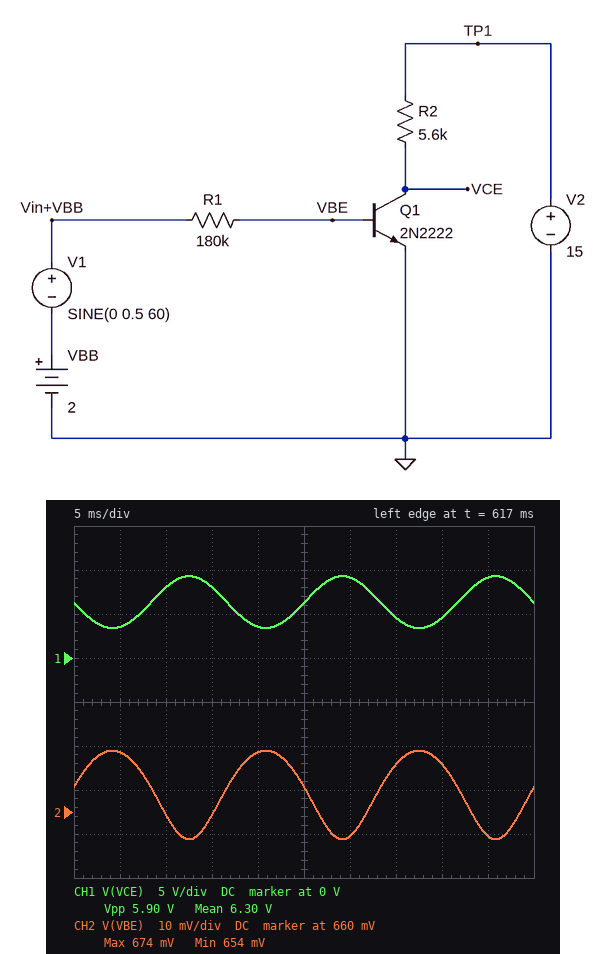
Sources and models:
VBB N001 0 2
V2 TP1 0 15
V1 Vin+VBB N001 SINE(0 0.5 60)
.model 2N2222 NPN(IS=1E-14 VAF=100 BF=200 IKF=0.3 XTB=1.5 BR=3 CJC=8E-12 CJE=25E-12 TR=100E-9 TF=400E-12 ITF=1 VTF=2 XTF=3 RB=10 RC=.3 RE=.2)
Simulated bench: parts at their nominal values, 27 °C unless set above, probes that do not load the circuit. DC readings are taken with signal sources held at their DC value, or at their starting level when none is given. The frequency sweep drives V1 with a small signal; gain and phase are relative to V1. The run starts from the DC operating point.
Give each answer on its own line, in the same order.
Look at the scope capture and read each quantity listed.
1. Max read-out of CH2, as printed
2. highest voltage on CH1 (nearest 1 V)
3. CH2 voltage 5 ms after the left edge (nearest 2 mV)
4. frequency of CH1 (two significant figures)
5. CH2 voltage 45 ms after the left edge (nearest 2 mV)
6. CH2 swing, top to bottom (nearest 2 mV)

674 mV
9 V
674 mV
60 Hz
654 mV
20 mV
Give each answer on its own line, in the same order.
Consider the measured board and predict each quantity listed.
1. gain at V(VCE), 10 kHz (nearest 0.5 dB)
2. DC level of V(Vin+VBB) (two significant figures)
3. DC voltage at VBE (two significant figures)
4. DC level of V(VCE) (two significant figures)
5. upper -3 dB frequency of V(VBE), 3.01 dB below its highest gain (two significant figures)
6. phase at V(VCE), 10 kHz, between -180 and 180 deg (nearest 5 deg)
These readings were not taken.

15.0 dB
2.0 V
670 mV
6.3 V
36 kHz
165 deg
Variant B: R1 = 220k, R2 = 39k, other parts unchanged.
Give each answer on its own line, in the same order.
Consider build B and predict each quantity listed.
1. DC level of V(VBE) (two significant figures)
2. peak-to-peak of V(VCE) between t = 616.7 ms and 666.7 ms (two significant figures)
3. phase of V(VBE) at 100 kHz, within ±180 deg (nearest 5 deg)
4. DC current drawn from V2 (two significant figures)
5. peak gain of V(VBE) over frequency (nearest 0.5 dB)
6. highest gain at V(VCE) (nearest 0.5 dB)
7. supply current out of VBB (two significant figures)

630 mV
29 mV
-10 deg
380 µA
-58.0 dB
-31.5 dB
6.2 µA
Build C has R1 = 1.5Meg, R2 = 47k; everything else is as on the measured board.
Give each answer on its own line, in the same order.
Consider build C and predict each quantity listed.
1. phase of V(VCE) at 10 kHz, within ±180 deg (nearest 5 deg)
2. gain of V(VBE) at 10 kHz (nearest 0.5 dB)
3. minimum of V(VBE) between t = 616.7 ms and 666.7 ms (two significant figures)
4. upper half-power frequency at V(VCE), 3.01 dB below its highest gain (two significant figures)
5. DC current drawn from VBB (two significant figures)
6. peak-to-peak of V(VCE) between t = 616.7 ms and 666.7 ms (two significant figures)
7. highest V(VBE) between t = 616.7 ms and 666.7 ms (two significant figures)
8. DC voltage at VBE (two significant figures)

115 deg
-43.0 dB
600 mV
4.3 kHz
930 nA
5.9 V
620 mV
610 mV
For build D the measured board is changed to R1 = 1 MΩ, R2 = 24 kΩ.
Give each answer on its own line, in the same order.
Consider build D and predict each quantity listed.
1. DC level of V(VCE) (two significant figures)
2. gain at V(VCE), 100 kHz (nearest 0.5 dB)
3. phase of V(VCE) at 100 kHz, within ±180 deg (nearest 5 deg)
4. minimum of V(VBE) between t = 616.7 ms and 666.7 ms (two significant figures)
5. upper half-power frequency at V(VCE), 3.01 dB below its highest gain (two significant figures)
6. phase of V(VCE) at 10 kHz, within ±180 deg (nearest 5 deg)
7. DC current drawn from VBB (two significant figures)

7.9 V
-7.5 dB
95 deg
610 mV
8.7 kHz
130 deg
1.4 µA
